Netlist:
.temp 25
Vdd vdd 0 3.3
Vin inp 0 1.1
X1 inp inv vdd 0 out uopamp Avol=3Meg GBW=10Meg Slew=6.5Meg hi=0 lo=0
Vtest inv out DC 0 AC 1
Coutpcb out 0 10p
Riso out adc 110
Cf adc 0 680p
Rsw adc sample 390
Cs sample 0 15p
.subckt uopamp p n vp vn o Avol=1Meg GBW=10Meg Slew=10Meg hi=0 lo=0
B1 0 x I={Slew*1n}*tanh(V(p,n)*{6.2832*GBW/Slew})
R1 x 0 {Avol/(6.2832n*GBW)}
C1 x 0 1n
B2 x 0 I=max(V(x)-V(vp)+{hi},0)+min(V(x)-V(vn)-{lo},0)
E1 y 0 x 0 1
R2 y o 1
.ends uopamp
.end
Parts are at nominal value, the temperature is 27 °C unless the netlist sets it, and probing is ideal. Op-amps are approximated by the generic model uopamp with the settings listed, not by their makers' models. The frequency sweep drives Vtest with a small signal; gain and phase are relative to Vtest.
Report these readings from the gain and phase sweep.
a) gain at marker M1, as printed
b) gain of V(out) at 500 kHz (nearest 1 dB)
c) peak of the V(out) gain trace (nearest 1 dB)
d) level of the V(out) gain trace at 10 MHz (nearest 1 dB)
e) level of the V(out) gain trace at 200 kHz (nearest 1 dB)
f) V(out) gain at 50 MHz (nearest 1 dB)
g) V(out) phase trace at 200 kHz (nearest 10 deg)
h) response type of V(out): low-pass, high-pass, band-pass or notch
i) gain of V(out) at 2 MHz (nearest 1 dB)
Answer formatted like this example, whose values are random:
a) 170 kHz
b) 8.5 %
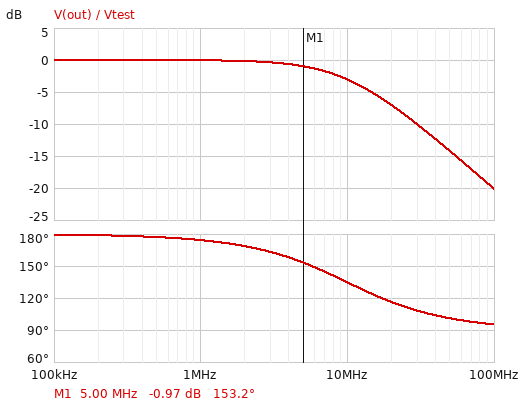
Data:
a) -0.97 dB
b) 0 dB
c) 0 dB
d) -3 dB
e) 0 dB
f) -14 dB
g) 180 deg
h) low-pass
i) 0 dB
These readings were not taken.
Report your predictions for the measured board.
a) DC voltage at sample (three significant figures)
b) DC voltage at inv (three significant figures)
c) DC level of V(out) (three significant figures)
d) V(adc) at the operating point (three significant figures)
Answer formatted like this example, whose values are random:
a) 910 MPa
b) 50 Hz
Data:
a) 1.10 V
b) 1.10 V
c) 1.10 V
d) 1.10 V
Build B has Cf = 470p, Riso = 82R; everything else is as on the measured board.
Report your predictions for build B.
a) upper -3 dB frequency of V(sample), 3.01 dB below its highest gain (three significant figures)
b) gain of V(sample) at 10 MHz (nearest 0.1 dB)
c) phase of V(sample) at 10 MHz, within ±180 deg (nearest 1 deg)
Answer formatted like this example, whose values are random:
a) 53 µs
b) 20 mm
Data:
a) 3.48 MHz
b) -12.2 dB
c) 47 deg
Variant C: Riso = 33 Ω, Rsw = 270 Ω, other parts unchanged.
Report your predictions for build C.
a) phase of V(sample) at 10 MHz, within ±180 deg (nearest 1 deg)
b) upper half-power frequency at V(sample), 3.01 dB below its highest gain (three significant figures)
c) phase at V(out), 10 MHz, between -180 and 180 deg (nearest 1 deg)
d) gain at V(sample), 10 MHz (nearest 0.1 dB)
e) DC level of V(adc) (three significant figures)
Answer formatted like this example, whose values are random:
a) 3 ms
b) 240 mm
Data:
a) 65 deg
b) 5.18 MHz
c) 134 deg
d) -8.2 dB
e) 1.10 V
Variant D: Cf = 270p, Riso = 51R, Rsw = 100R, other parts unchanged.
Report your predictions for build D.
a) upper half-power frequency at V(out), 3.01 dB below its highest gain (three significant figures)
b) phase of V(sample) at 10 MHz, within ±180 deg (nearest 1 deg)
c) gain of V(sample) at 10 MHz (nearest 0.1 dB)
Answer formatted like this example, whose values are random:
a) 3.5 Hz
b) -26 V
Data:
a) 10.0 MHz
b) 87 deg
c) -5.7 dB
